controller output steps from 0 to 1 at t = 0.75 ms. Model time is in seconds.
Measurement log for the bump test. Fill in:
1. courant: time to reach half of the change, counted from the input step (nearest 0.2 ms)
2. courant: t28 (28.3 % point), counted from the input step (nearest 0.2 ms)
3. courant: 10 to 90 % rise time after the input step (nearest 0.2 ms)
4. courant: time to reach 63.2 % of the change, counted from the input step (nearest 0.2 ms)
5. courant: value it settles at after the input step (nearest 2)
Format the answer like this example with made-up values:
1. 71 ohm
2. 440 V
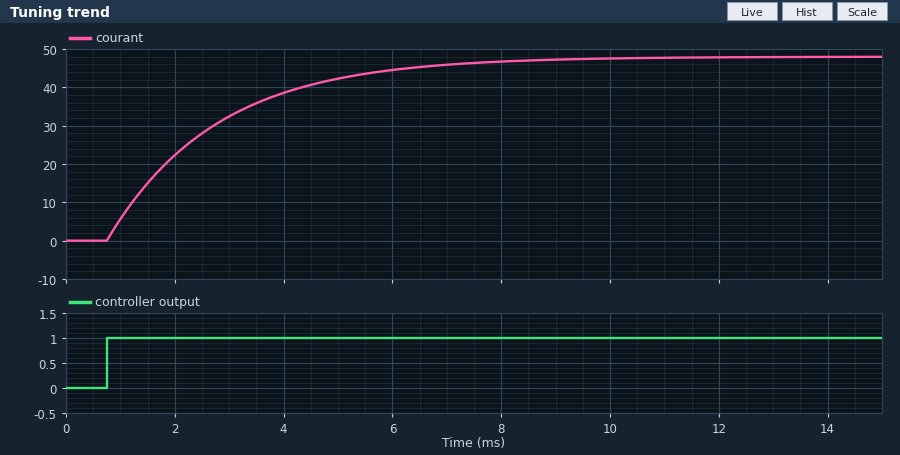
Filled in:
1. 1.4 ms
2. 0.6 ms
3. 4.4 ms
4. 2.0 ms
5. 48
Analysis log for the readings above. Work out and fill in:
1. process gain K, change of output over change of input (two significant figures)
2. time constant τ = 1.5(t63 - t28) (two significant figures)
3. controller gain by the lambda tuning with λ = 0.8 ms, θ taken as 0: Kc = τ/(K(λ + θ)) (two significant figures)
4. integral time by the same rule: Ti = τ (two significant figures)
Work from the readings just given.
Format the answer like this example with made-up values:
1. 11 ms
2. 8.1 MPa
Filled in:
1. 48
2. 2.1 ms
3. 0.055
4. 2.1 ms
